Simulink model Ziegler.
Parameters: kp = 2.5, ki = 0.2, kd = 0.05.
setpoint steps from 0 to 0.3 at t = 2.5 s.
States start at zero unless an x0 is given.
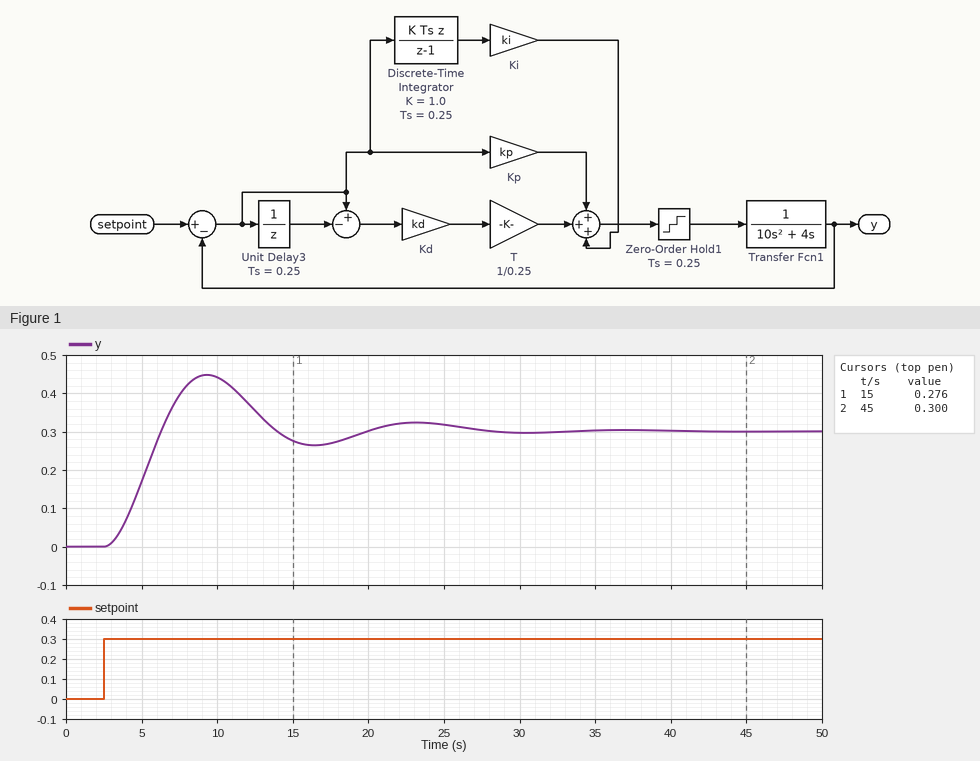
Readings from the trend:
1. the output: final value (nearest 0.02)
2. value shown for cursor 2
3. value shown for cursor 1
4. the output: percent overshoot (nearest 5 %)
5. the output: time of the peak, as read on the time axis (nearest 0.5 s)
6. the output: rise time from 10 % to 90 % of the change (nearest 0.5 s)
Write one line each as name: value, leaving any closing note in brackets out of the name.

the output: final value: 0.30
value shown for cursor 2: 0.300
value shown for cursor 1: 0.276
the output: percent overshoot: 50 %
the output: time of the peak, as read on the time axis: 9.5 s
the output: rise time from 10 % to 90 % of the change: 2.5 s
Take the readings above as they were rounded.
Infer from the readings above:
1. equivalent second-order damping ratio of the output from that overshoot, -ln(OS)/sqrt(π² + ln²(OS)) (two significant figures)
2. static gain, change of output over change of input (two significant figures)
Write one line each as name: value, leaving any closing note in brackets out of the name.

equivalent second-order damping ratio of the output from that overshoot, -ln(OS)/sqrt(π² + ln²(OS)): 0.22
static gain, change of output over change of input: 1.0
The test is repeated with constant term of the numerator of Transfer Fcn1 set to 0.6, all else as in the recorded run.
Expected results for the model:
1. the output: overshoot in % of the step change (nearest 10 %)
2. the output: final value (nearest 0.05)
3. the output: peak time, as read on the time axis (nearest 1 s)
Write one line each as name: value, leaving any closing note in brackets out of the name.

the output: overshoot in % of the step change: 40 %
the output: final value: 0.30
the output: peak time, as read on the time axis: 12 s
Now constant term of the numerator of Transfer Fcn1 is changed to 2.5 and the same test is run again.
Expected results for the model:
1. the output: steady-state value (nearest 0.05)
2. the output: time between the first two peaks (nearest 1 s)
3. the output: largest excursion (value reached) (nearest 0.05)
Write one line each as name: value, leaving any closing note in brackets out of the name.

the output: steady-state value: 0.30
the output: time between the first two peaks: 8 s
the output: largest excursion (value reached): 0.50
